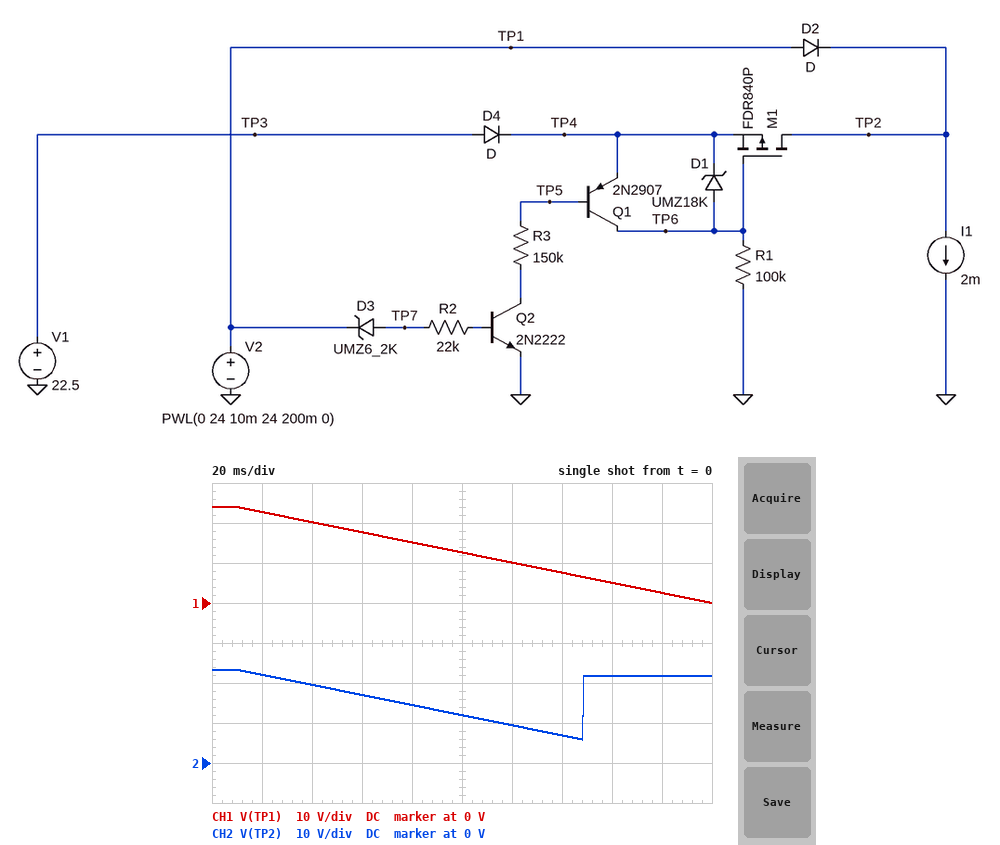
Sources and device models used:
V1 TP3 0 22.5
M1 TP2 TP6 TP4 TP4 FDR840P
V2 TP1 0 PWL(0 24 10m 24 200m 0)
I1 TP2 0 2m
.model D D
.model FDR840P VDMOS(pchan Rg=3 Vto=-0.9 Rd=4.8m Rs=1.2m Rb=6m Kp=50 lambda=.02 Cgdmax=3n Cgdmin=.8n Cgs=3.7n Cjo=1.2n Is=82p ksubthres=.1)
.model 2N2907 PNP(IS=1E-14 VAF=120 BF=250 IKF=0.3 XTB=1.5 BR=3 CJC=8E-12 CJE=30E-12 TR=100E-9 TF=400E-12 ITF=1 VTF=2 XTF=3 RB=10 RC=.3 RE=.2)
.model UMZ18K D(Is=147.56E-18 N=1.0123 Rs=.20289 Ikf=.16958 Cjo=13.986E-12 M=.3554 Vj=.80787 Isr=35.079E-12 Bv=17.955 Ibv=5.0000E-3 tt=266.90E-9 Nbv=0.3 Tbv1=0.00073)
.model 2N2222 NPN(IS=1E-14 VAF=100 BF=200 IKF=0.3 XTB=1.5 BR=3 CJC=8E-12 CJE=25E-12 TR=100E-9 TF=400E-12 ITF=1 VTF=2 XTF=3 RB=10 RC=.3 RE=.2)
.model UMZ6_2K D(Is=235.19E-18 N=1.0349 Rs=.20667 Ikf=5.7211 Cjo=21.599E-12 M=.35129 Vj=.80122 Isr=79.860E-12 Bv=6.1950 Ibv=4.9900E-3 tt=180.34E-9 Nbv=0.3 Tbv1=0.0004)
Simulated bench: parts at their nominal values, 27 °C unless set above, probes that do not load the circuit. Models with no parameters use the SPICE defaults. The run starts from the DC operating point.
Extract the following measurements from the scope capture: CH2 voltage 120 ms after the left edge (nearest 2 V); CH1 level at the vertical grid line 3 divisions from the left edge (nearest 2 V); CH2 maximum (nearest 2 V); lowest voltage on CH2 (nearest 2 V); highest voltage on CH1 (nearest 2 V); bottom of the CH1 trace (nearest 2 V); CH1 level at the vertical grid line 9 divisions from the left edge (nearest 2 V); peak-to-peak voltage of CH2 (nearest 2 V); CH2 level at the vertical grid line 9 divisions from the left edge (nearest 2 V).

10 V
18 V
24 V
6 V
24 V
0 V
2 V
18 V
22 V
